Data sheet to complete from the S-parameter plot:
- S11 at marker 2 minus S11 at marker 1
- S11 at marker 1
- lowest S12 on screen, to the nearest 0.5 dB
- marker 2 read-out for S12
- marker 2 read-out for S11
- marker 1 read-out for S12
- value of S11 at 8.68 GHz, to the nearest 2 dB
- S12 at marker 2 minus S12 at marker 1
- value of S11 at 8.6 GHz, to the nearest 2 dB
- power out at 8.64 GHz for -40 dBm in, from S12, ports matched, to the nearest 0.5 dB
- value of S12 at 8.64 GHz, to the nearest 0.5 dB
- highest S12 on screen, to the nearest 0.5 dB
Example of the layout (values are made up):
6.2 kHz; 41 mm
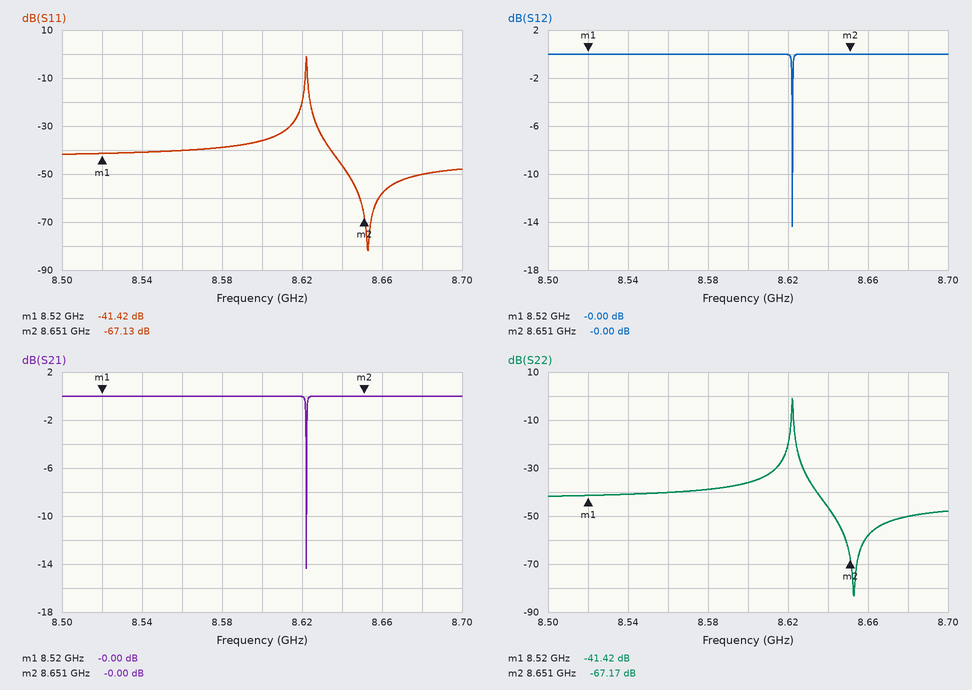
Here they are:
-25.71 dB; -41.42 dB; -14.5 dB; -0.00 dB; -67.13 dB; -0.00 dB; -50 dB; 0.00 dB; -36 dB; -40.0 dBm; 0.0 dB; 0.0 dB
